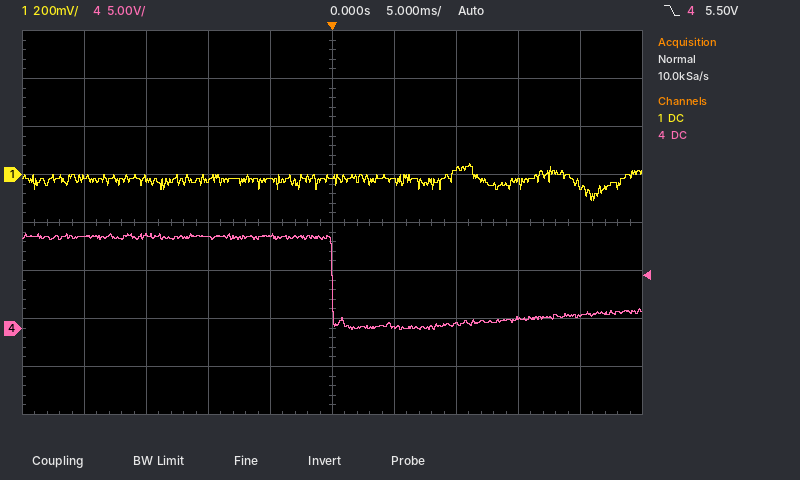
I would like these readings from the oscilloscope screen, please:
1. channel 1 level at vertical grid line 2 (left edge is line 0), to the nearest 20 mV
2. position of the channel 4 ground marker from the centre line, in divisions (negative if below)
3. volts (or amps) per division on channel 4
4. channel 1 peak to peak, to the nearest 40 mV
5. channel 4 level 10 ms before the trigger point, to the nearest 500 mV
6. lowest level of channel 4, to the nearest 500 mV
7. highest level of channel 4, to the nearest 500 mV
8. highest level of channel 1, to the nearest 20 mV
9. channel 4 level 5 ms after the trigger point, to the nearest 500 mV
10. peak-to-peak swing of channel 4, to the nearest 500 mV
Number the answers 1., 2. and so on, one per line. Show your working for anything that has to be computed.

1. -20 mV
2. -2.2 div
3. 5 V
4. 160 mV
5. 9.5 V
6. 0.0 V
7. 10.0 V
8. 40 mV
9. 0.0 V
10. 10.0 V − (0.0 V) = 10.0 V
